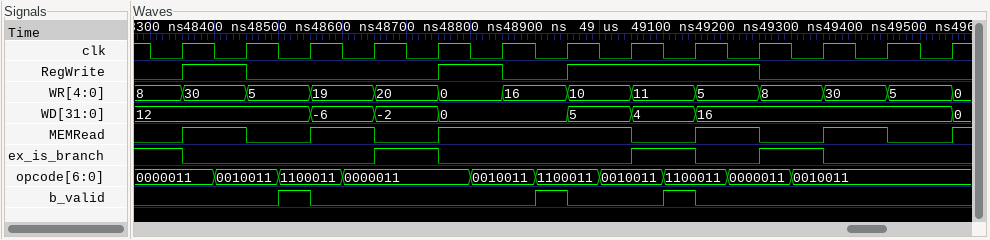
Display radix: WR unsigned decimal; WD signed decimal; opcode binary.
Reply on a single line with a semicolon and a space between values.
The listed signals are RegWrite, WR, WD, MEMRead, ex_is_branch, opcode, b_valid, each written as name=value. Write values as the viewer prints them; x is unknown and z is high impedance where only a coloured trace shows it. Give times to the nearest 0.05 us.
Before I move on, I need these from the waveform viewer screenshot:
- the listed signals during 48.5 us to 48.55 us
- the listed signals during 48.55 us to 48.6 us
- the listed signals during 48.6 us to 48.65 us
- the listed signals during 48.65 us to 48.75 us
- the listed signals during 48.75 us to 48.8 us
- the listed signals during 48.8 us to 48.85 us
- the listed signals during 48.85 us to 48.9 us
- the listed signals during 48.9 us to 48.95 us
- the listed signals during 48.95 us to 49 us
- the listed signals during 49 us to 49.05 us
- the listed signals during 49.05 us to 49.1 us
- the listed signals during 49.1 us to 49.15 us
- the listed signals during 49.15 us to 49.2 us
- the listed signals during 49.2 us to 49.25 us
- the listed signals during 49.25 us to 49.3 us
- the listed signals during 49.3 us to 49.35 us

RegWrite=0, WR=5, WD=12, MEMRead=0, ex_is_branch=0, opcode=1100011, b_valid=1; RegWrite=0, WR=19, WD=-6, MEMRead=1, ex_is_branch=0, opcode=1100011, b_valid=0; RegWrite=0, WR=19, WD=-6, MEMRead=1, ex_is_branch=0, opcode=0000011, b_valid=0; RegWrite=0, WR=20, WD=-2, MEMRead=0, ex_is_branch=1, opcode=0000011, b_valid=0; RegWrite=1, WR=0, WD=0, MEMRead=1, ex_is_branch=0, opcode=0000011, b_valid=0; RegWrite=1, WR=0, WD=0, MEMRead=1, ex_is_branch=0, opcode=0010011, b_valid=0; RegWrite=0, WR=16, WD=0, MEMRead=1, ex_is_branch=0, opcode=0010011, b_valid=0; RegWrite=0, WR=16, WD=0, MEMRead=1, ex_is_branch=0, opcode=1100011, b_valid=1; RegWrite=1, WR=10, WD=5, MEMRead=1, ex_is_branch=0, opcode=1100011, b_valid=0; RegWrite=1, WR=10, WD=5, MEMRead=1, ex_is_branch=0, opcode=0010011, b_valid=0; RegWrite=1, WR=11, WD=4, MEMRead=0, ex_is_branch=1, opcode=0010011, b_valid=0; RegWrite=1, WR=11, WD=4, MEMRead=0, ex_is_branch=1, opcode=1100011, b_valid=1; RegWrite=1, WR=5, WD=16, MEMRead=1, ex_is_branch=0, opcode=1100011, b_valid=0; RegWrite=1, WR=5, WD=16, MEMRead=1, ex_is_branch=0, opcode=0000011, b_valid=0; RegWrite=0, WR=8, WD=16, MEMRead=0, ex_is_branch=1, opcode=0000011, b_valid=0; RegWrite=0, WR=8, WD=16, MEMRead=0, ex_is_branch=1, opcode=0010011, b_valid=0
